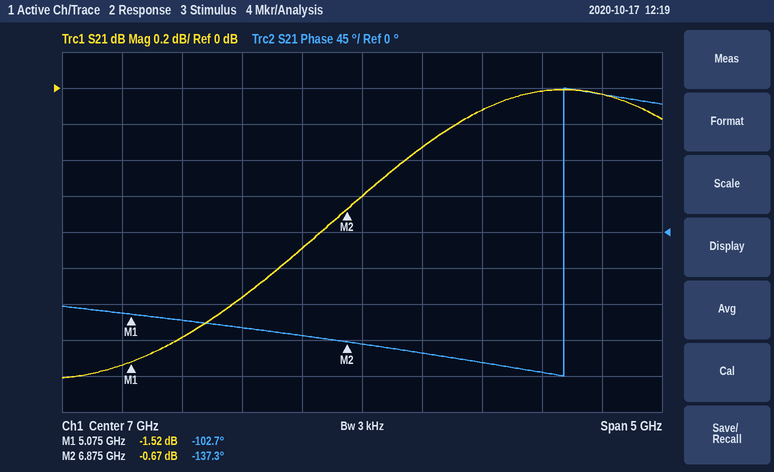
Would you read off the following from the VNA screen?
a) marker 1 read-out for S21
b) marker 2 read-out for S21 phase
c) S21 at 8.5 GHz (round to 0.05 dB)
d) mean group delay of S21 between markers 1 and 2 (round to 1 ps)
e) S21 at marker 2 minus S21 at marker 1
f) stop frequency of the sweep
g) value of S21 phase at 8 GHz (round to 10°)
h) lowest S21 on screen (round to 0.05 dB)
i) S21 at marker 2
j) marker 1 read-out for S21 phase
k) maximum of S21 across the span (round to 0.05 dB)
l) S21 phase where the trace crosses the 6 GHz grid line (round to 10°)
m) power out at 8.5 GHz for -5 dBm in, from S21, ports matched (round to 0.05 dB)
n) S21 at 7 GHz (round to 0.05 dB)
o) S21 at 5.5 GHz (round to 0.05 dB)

-1.52 dB
-137.3°
0.00 dB
53 ps
0.85 dB
9.5 GHz
-160°
-1.60 dB
-0.67 dB
-102.7°
0.00 dB
-120°
-5.00 dBm
-0.60 dB
-1.40 dB
